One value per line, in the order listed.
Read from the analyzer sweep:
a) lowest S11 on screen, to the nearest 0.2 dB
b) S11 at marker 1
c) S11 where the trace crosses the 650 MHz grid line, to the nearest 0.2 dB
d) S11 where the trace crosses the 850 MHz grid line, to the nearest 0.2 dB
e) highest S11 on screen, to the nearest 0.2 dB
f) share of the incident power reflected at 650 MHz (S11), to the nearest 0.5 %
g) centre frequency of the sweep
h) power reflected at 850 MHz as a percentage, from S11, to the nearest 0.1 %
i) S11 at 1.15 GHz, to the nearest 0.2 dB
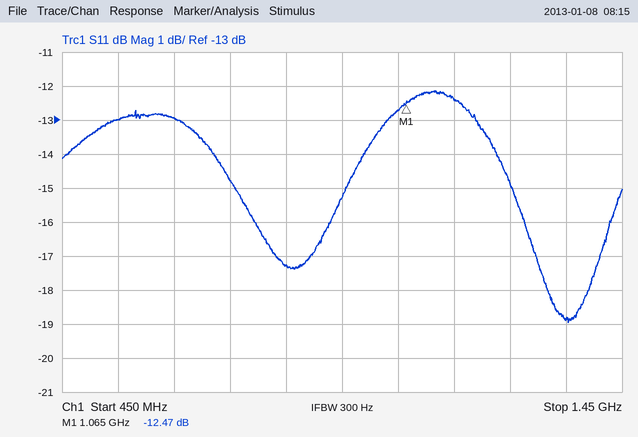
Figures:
-19.0 dB
-12.47 dB
-13.0 dB
-17.2 dB
-12.2 dB
5.0 %
950 MHz
1.9 %
-12.4 dB
